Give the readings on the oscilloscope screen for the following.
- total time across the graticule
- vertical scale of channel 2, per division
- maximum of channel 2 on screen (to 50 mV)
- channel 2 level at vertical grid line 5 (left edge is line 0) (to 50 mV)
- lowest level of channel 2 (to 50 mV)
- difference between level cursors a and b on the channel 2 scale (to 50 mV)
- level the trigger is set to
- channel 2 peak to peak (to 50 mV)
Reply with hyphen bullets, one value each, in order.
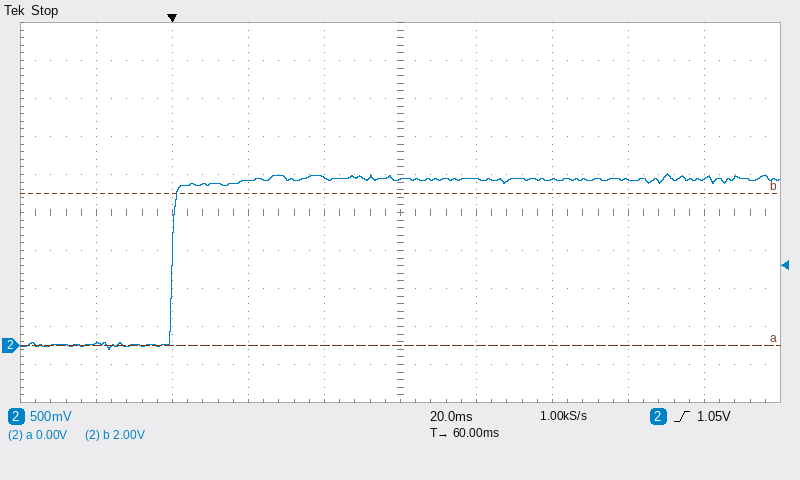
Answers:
- 200 ms
- 500 mV
- 2.25 V
- 2.20 V
- -50 mV
- 2.00 V
- 1.05 V
- 2.30 V
